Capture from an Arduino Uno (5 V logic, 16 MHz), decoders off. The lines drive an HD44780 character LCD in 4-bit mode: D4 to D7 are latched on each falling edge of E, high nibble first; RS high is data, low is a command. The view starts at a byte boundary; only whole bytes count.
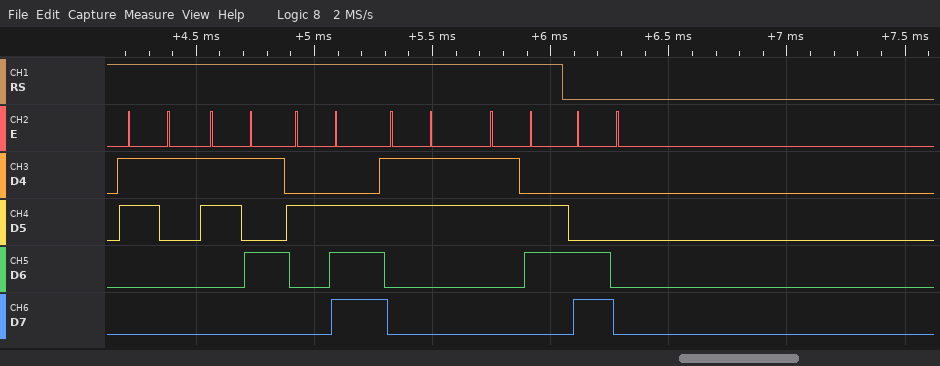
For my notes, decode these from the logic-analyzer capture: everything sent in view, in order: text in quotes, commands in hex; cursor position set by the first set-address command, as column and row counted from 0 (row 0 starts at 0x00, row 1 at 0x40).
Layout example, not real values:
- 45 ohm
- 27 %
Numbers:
- "15.36" 0xC0
- column 0, row 1
